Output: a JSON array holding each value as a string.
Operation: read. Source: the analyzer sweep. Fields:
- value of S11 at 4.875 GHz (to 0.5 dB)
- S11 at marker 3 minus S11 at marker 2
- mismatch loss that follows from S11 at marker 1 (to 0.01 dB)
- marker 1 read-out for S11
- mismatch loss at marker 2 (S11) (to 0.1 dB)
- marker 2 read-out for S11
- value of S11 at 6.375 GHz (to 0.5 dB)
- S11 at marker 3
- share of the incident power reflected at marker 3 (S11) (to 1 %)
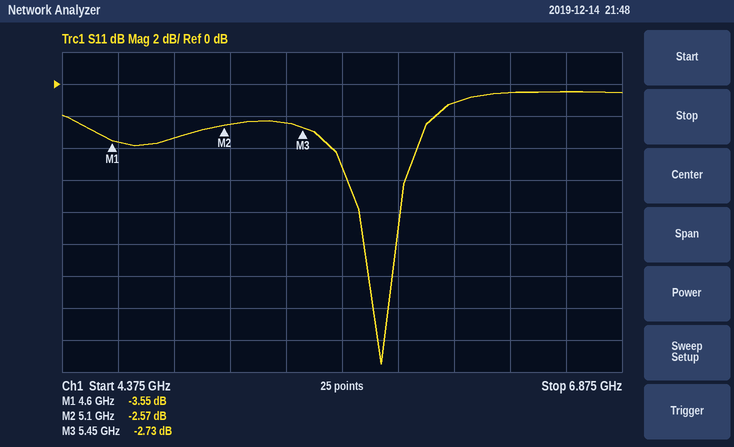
["-3.5 dB", "-0.16 dB", "2.53 dB", "-3.55 dB", "3.5 dB", "-2.57 dB", "-0.5 dB", "-2.73 dB", "53 %"]
